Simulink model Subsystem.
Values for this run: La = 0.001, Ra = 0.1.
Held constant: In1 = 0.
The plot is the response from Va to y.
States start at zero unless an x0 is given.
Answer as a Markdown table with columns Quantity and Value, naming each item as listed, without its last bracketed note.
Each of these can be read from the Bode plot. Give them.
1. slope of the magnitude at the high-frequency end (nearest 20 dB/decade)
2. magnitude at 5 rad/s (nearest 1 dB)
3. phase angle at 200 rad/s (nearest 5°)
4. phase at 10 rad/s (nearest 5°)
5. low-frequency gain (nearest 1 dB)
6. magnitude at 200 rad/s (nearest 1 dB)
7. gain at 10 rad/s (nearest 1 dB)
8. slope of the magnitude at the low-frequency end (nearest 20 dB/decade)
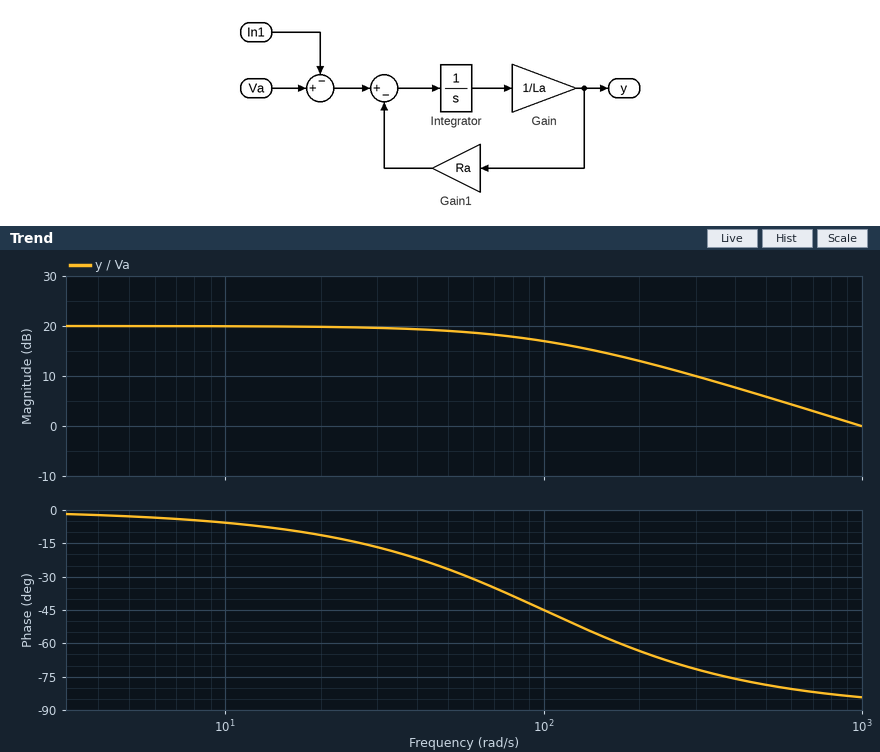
| Quantity | Value |
|---|---|
| slope of the magnitude at the high-frequency end | -20 dB/decade |
| magnitude at 5 rad/s | 20 dB |
| phase angle at 200 rad/s | -65° |
| phase at 10 rad/s | -5° |
| low-frequency gain | 20 dB |
| magnitude at 200 rad/s | 13 dB |
| gain at 10 rad/s | 20 dB |
| slope of the magnitude at the low-frequency end | 0 dB/decade |
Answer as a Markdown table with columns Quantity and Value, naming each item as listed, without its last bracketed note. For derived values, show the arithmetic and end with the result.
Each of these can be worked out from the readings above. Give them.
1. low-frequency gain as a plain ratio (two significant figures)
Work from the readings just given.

| Quantity | Value |
|---|---|
| low-frequency gain as a plain ratio | 10^(20 / 20) = 10 |
